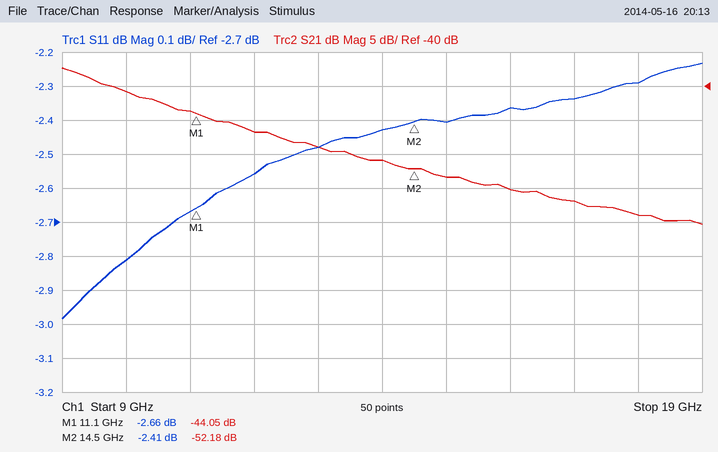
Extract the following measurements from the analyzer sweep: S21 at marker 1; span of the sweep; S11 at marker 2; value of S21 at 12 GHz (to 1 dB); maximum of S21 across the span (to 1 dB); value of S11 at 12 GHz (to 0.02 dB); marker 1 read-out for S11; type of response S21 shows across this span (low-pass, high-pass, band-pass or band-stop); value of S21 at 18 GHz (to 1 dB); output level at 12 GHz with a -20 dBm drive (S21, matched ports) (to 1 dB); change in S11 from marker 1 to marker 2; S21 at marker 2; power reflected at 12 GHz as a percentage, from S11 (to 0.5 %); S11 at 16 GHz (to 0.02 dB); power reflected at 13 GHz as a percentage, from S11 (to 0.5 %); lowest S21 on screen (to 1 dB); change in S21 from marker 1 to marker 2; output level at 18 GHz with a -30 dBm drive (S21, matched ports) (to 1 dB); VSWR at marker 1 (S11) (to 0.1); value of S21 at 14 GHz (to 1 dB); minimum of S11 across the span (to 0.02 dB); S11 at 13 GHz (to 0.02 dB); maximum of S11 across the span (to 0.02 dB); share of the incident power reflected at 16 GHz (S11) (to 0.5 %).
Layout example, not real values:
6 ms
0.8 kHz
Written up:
-44.05 dB
10 GHz
-2.41 dB
-47 dB
-37 dB
-2.56 dB
-2.66 dB
low-pass
-59 dB
-67 dBm
0.25 dB
-52.18 dB
55.5 %
-2.36 dB
56.5 %
-60 dB
-8.13 dB
-89 dBm
6.6
-51 dB
-2.98 dB
-2.48 dB
-2.24 dB
58.0 %
